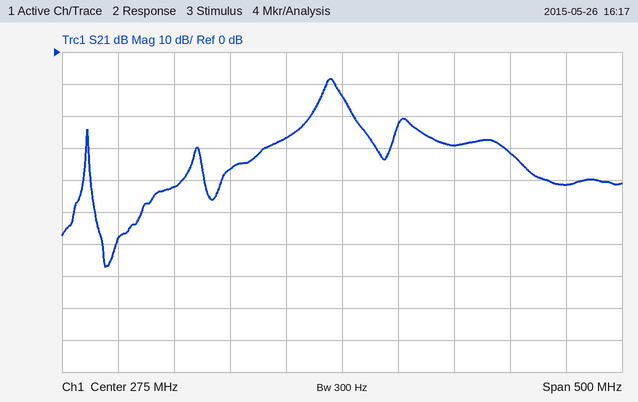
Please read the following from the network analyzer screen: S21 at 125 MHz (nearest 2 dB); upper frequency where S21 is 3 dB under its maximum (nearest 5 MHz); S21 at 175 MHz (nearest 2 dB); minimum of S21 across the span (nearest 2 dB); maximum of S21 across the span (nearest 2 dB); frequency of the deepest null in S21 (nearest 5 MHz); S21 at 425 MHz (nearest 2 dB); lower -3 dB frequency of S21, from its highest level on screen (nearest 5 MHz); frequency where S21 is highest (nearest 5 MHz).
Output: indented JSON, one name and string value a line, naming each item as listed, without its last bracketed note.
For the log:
{
  "S21 at 125 MHz": "-42 dB",
  "upper frequency where S21 is 3 dB under its maximum": "270 MHz",
  "S21 at 175 MHz": "-36 dB",
  "minimum of S21 across the span": "-68 dB",
  "maximum of S21 across the span": "-8 dB",
  "frequency of the deepest null in S21": "65 MHz",
  "S21 at 425 MHz": "-32 dB",
  "lower -3 dB frequency of S21, from its highest level on screen": "260 MHz",
  "frequency where S21 is highest": "265 MHz"
}
